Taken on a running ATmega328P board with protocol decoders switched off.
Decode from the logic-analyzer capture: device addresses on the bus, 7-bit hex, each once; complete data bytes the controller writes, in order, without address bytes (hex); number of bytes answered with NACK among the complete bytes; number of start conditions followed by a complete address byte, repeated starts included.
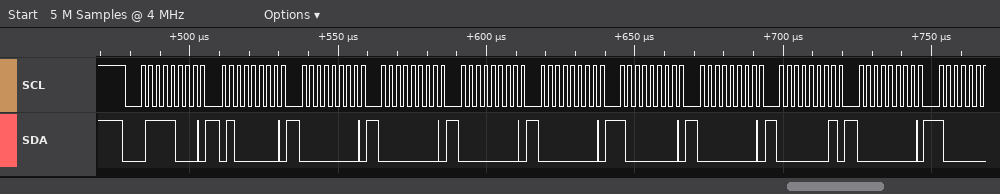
0x3C
40 00 00 00 00 80 00 01 00
0
1
